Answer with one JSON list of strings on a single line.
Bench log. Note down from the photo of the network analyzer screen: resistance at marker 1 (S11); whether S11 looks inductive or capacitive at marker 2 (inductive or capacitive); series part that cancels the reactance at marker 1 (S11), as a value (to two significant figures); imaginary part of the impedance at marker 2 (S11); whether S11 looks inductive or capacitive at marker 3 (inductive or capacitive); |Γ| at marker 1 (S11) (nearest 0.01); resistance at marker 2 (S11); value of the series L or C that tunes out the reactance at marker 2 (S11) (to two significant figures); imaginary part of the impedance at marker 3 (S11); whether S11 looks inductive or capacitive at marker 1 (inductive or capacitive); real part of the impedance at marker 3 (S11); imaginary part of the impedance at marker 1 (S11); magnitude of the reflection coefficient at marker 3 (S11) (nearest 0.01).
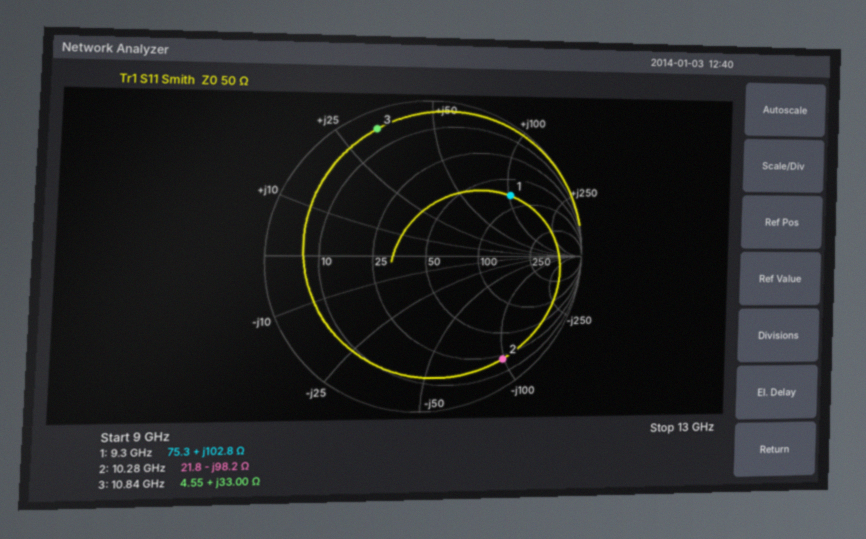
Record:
["75.3 Ω", "capacitive", "170 fF", "-98.2 Ω", "inductive", "0.65", "21.8 Ω", "1.5 nH", "+33.00 Ω", "inductive", "4.55 Ω", "+102.8 Ω", "0.88"]
